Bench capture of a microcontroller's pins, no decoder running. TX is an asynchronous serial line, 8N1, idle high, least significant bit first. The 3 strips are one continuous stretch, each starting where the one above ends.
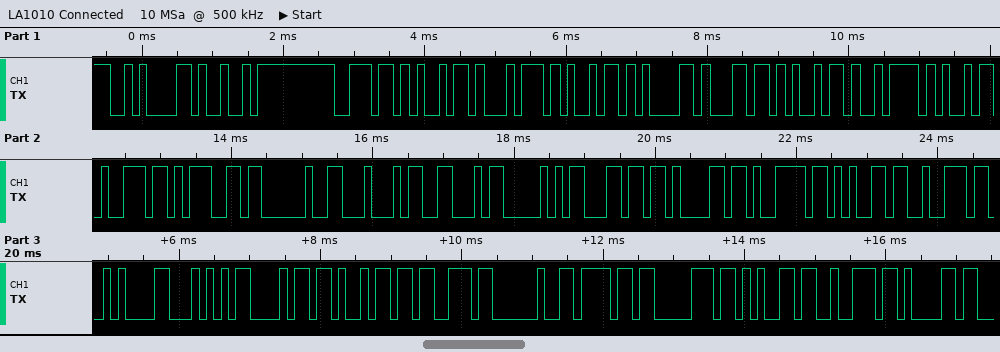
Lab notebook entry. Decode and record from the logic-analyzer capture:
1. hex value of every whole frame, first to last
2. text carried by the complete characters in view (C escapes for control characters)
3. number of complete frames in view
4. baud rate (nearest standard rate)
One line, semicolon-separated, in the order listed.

0A 49 6E 69 74 69 61 6C 69 7A 69 6E 67 20 44 46 50 6C 61 79 65 72 0A 54 68 69 73 20 6F 70 65 72 61; "\nInitializing DFPlayer\nThis opera"; 33; 9600 baud
